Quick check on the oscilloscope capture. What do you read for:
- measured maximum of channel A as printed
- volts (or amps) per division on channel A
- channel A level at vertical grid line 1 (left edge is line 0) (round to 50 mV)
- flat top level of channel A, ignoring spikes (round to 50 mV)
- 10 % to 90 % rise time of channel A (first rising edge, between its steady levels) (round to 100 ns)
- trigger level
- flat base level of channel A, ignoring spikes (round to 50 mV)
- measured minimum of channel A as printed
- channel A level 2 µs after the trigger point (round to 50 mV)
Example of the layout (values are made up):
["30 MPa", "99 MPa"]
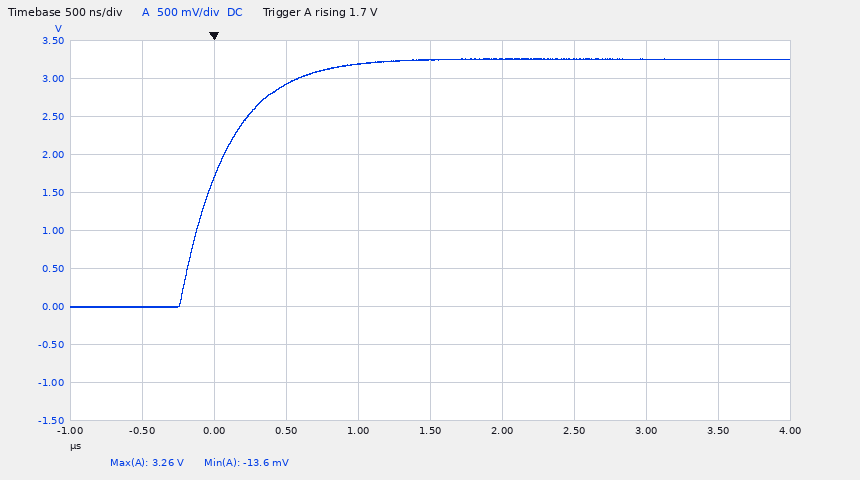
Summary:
["3.26 V", "500 mV", "0 mV", "3.25 V", "700 ns", "1.7 V", "0 mV", "-13.6 mV", "3.25 V"]
